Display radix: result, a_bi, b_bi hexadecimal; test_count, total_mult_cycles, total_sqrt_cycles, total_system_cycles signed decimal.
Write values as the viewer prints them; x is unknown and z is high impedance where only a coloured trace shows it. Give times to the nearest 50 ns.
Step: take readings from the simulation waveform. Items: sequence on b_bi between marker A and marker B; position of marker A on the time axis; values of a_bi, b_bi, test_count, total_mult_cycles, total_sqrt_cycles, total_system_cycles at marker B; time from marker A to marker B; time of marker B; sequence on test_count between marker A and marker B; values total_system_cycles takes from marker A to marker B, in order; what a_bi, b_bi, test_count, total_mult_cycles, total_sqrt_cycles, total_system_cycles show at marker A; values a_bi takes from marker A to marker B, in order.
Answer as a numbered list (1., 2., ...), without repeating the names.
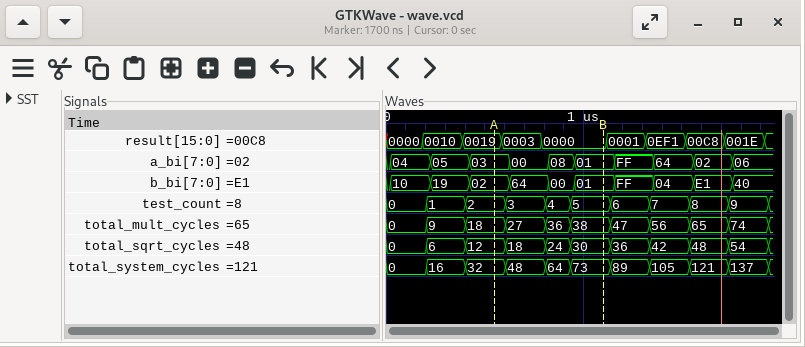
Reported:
1. 02, 64, 00, 01
2. 550 ns
3. a_bi=01, b_bi=01, test_count=5, total_mult_cycles=38, total_sqrt_cycles=30, total_system_cycles=73
4. 550 ns
5. 1100 ns
6. 2, 3, 4, 5
7. 32, 48, 64, 73
8. a_bi=03, b_bi=02, test_count=2, total_mult_cycles=18, total_sqrt_cycles=12, total_system_cycles=32
9. 03, 00, 08, 01
